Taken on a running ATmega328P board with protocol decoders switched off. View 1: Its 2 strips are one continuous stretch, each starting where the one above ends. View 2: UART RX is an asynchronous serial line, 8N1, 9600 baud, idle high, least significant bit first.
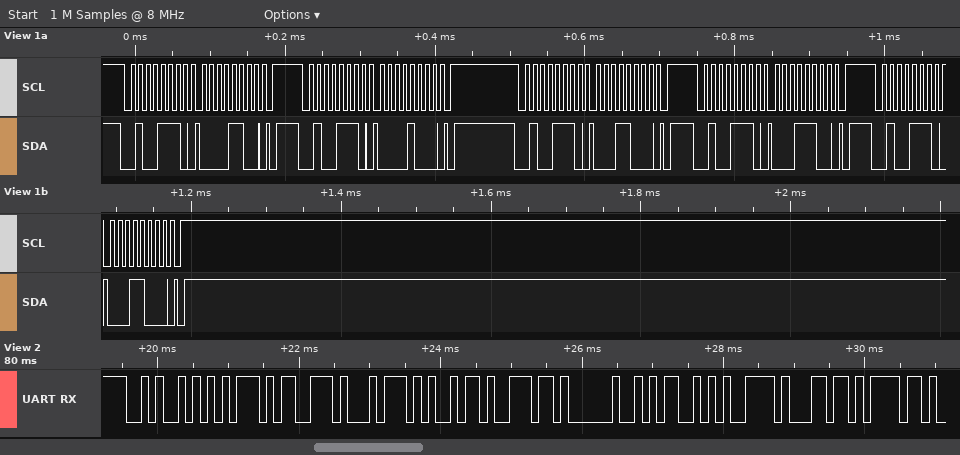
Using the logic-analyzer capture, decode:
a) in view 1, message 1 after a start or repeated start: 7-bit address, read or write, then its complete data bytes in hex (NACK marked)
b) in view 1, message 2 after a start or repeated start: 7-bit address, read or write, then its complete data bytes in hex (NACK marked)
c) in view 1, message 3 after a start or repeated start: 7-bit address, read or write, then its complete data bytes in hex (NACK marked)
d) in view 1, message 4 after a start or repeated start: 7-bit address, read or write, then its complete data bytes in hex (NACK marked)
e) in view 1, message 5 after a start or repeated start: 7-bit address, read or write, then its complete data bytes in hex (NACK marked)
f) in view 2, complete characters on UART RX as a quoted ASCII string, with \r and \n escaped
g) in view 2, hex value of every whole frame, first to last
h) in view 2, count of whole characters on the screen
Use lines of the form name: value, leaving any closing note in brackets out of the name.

in view 1, message 1 after a start or repeated start: 7-bit address, read or write, then its complete data bytes in hex: 0x27 write: 0C
in view 1, message 2 after a start or repeated start: 7-bit address, read or write, then its complete data bytes in hex: 0x27 write: 08
in view 1, message 3 after a start or repeated start: 7-bit address, read or write, then its complete data bytes in hex: 0x27 write: 18
in view 1, message 4 after a start or repeated start: 7-bit address, read or write, then its complete data bytes in hex: 0x27 write: 1C
in view 1, message 5 after a start or repeated start: 7-bit address, read or write, then its complete data bytes in hex: 0x27 write: 18
in view 2, complete characters on UART RX as a quoted ASCII string, with \r and \n escaped: "Justin Mylo"
in view 2, hex value of every whole frame, first to last: 0x4A 0x75 0x73 0x74 0x69 0x6E 0x20 0x4D 0x79 0x6C 0x6F
in view 2, count of whole characters on the screen: 11
